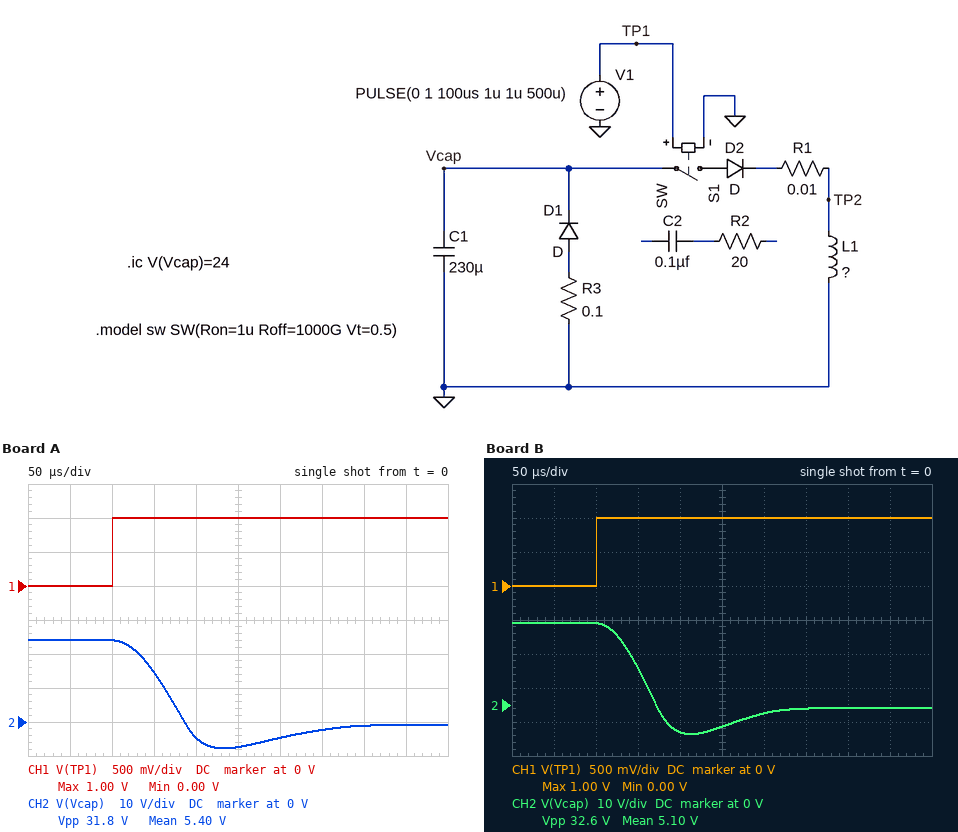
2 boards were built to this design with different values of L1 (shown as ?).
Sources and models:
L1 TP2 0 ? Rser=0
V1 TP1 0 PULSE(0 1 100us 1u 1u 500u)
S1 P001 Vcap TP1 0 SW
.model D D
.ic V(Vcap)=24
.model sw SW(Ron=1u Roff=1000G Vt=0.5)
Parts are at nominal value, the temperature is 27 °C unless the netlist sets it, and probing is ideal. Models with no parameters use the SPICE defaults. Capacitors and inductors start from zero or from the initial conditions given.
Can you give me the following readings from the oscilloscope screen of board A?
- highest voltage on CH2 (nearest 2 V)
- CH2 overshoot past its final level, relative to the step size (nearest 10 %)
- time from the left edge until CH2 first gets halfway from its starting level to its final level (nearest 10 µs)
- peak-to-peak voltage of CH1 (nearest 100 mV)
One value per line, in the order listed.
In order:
24 V
30 %
160 µs
1.0 V
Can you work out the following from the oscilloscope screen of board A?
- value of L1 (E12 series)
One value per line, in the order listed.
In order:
12 µH
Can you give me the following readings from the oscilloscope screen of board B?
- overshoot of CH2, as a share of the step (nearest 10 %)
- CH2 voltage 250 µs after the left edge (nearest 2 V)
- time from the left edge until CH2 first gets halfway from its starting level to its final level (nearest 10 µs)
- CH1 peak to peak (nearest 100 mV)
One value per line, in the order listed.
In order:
30 %
-6 V
150 µs
1.0 V
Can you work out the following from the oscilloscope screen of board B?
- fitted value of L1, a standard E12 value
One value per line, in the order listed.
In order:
8.2 µH
